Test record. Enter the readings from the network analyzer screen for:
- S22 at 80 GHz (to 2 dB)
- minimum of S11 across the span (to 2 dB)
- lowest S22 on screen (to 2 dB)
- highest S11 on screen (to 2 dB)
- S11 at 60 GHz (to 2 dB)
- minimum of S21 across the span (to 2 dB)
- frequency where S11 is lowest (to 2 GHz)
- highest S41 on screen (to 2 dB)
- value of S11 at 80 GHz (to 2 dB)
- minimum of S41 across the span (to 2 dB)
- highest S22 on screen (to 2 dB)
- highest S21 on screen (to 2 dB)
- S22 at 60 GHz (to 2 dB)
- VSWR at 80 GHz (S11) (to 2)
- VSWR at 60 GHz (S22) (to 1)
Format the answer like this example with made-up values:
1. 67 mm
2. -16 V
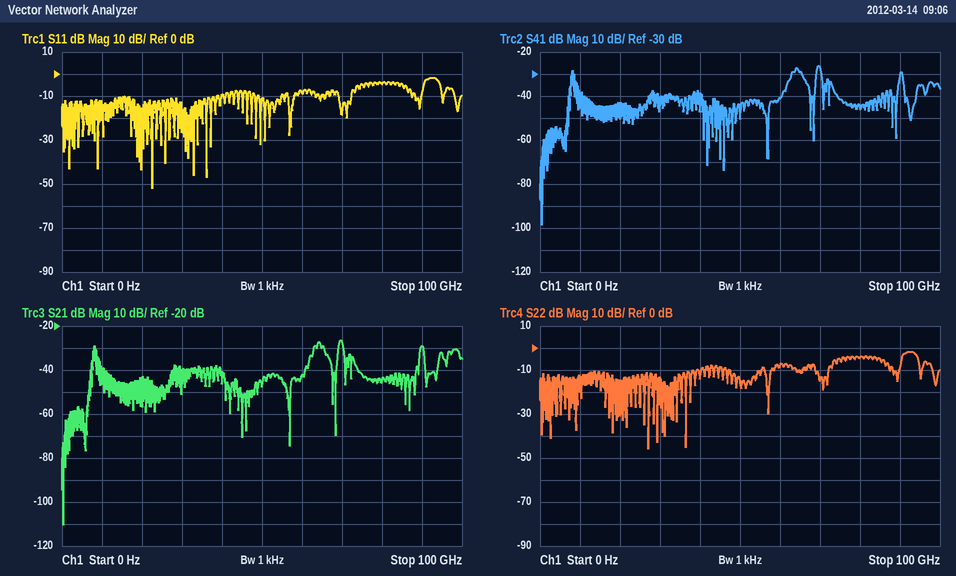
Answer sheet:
1. -4 dB
2. -52 dB
3. -46 dB
4. -2 dB
5. -8 dB
6. -110 dB
7. 22 GHz
8. -26 dB
9. -4 dB
10. -98 dB
11. -2 dB
12. -26 dB
13. -8 dB
14. 4
15. 2
